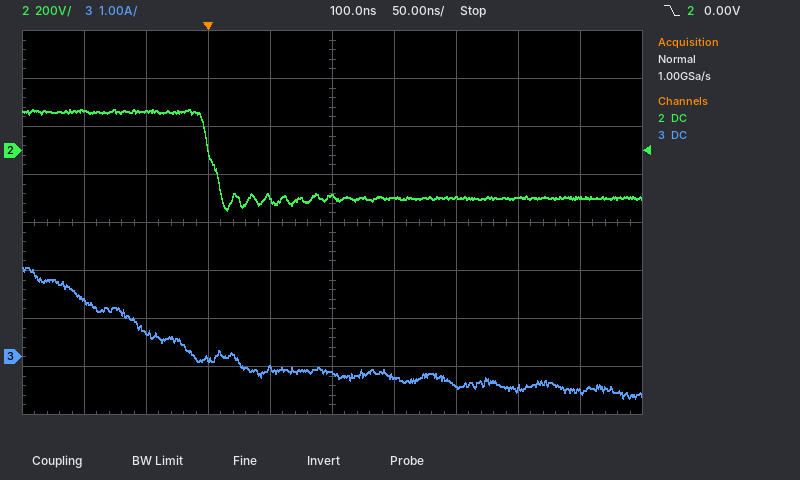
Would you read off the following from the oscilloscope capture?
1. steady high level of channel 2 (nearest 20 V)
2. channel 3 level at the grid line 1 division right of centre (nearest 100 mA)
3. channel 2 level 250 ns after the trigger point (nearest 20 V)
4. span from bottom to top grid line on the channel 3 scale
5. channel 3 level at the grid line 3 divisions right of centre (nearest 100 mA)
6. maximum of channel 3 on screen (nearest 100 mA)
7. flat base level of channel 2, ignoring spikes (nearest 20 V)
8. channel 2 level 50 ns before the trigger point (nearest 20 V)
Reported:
160 V
-400 mA
-200 V
8 A
-700 mA
1.9 A
-200 V
160 V
